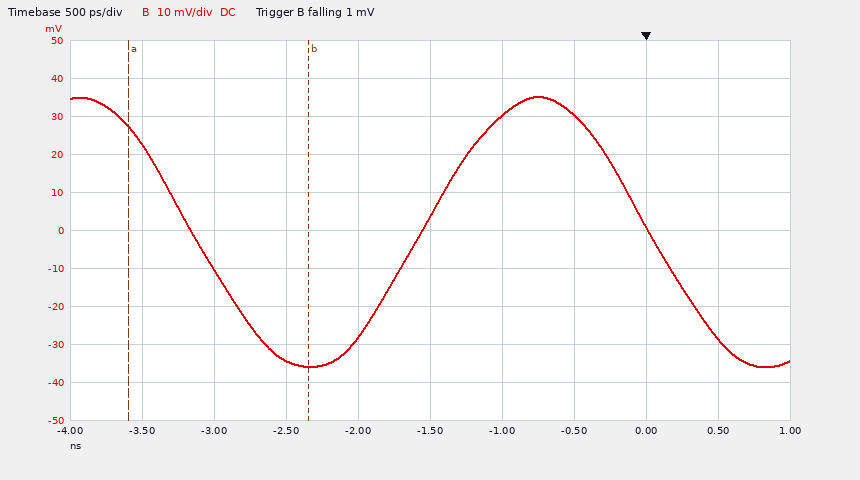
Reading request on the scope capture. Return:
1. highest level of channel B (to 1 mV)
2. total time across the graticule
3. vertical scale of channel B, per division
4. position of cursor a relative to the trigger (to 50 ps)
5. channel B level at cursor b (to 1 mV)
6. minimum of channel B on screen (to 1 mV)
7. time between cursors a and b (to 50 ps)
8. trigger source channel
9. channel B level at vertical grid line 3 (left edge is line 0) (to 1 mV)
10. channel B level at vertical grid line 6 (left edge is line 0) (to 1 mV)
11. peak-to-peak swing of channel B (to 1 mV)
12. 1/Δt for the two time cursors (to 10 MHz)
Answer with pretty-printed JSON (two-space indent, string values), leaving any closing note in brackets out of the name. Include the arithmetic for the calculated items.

{
  "highest level of channel B": "35 mV",
  "total time across the graticule": "5 ns",
  "vertical scale of channel B, per division": "10 mV",
  "position of cursor a relative to the trigger": "-3.60 ns",
  "channel B level at cursor b": "-36 mV",
  "minimum of channel B on screen": "-36 mV",
  "time between cursors a and b": "1.25 ns",
  "trigger source channel": "channel B",
  "channel B level at vertical grid line 3 (left edge is line 0)": "-34 mV",
  "channel B level at vertical grid line 6 (left edge is line 0)": "30 mV",
  "peak-to-peak swing of channel B": "35 mV − (-36 mV) = 71 mV",
  "1/Δt for the two time cursors": "1 / 1.25 ns ≈ 800 MHz"
}
